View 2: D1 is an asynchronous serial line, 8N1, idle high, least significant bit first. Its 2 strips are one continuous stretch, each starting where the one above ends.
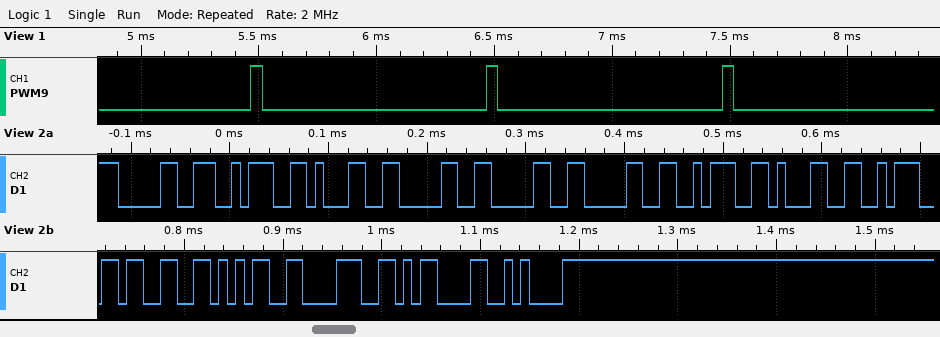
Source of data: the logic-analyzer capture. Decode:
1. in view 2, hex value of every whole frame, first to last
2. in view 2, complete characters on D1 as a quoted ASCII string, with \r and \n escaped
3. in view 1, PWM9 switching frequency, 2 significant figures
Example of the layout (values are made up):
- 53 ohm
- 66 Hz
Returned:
- 0x30 0x3A 0x31 0x30 0x30 0x30 0x3A 0x31 0x3A 0x33 0x35 0x38 0x0D 0x0A
- "0:1000:1:358\r\n"
- 1.0 kHz
